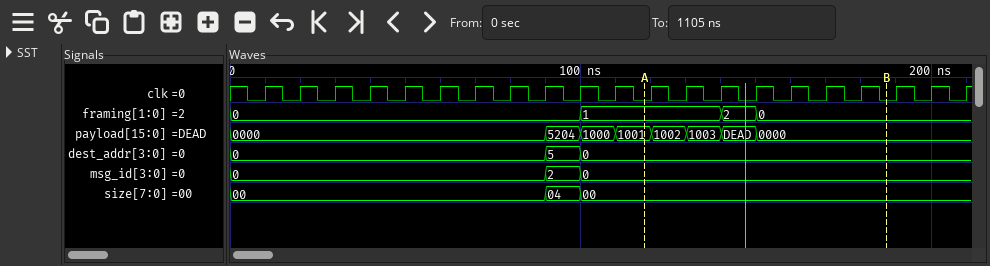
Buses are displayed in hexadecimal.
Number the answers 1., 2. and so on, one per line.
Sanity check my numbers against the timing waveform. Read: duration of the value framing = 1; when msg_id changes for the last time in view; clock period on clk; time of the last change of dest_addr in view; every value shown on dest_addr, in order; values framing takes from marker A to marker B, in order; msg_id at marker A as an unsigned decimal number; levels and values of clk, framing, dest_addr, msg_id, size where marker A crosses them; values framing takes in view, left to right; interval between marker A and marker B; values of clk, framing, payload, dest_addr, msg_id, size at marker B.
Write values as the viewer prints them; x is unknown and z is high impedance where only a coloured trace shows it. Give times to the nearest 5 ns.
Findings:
1. 40 ns
2. 100 ns
3. 10 ns
4. 100 ns
5. 0, 5, 0
6. 1, 2, 0
7. 0
8. clk=0, framing=1, dest_addr=0, msg_id=0, size=00
9. 0, 1, 2, 0
10. 70 ns
11. clk=0, framing=0, payload=0000, dest_addr=0, msg_id=0, size=00
